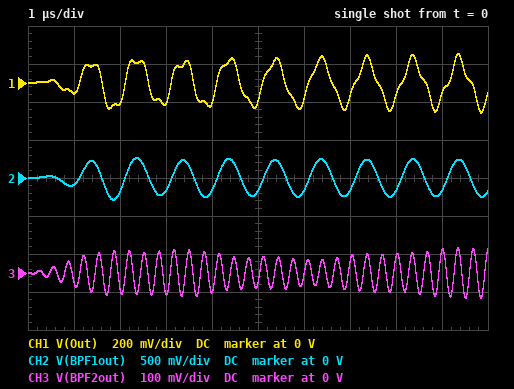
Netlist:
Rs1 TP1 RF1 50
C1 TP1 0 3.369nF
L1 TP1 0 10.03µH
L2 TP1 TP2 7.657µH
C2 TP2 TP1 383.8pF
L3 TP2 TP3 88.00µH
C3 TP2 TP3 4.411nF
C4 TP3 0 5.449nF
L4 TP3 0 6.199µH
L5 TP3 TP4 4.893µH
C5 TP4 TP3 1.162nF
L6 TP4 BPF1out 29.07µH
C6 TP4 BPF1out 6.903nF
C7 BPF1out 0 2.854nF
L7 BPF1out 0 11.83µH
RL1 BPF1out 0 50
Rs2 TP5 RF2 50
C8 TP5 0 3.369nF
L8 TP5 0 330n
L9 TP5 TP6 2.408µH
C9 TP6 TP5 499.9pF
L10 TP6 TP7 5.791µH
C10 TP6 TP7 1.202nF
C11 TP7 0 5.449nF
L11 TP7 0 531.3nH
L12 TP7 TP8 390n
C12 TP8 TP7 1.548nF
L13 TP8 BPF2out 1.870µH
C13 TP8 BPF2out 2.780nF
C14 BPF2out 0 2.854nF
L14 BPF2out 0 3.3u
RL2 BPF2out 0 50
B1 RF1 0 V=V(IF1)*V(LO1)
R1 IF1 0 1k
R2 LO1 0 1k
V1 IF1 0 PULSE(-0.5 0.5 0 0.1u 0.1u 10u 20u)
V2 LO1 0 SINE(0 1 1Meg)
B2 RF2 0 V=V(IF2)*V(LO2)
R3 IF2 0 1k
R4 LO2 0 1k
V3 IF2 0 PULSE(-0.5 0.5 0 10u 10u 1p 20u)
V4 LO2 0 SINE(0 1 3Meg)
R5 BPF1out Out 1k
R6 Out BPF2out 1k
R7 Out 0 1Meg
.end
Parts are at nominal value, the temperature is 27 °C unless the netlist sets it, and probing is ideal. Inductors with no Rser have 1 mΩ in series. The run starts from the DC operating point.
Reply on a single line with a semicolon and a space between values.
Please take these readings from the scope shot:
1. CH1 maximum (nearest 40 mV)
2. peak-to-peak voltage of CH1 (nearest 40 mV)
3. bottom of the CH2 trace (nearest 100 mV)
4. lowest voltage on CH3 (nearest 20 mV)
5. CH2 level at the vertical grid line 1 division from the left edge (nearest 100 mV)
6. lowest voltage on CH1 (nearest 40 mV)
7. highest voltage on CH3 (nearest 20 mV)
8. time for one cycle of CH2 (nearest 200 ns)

160 mV; 320 mV; -300 mV; -60 mV; -100 mV; -160 mV; 60 mV; 1.0 µs
